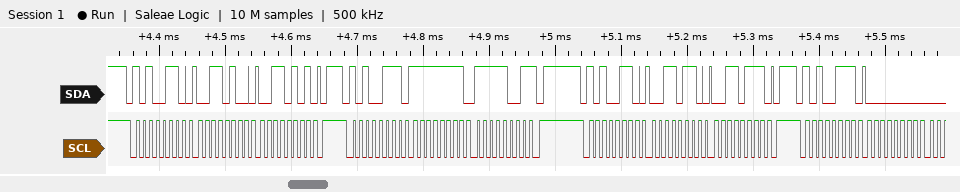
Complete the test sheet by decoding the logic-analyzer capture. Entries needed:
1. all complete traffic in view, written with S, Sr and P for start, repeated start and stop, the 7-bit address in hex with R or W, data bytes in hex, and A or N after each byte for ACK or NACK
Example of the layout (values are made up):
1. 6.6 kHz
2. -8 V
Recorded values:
1. S 53W A 34 A 35 A P S 53R A FF A F9 N P S 53W A 36 A 37 A P S 53R A 00 A
